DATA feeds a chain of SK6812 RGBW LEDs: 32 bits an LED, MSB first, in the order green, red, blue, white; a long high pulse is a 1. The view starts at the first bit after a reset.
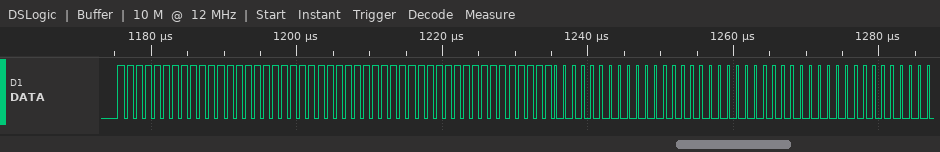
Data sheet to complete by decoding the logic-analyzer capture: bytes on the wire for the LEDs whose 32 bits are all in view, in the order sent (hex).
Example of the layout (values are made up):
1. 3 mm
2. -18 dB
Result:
1. FF FF FF FF FF FF 00 00
